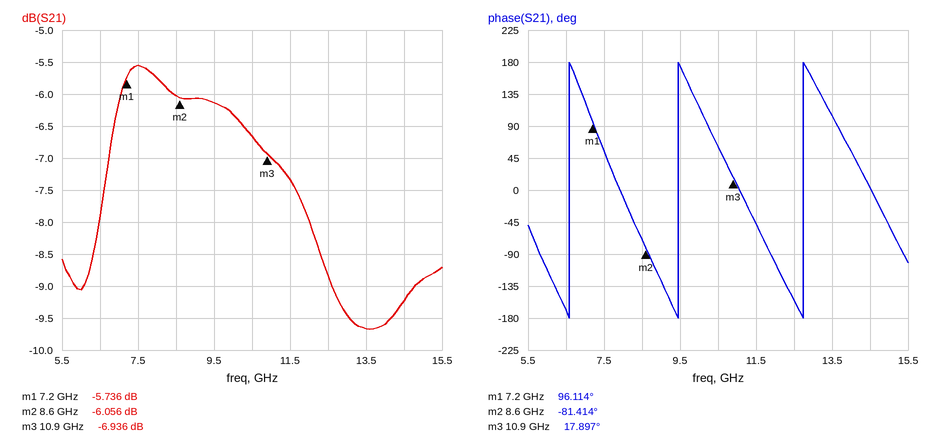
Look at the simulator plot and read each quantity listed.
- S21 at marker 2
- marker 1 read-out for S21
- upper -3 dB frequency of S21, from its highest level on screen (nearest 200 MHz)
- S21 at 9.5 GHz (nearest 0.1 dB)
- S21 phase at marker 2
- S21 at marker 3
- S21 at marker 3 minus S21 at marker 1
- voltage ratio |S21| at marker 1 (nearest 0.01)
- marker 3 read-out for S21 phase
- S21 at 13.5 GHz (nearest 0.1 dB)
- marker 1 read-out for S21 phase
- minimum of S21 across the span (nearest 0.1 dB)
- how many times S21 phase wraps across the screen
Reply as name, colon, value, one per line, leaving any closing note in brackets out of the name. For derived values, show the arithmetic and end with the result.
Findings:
S21 at marker 2: -6.056 dB
marker 1 read-out for S21: -5.736 dB
upper -3 dB frequency of S21, from its highest level on screen: 12.4 GHz
S21 at 9.5 GHz: -6.1 dB
S21 phase at marker 2: -81.414°
S21 at marker 3: -6.936 dB
S21 at marker 3 minus S21 at marker 1: -6.936 − (-5.736) = -1.200 dB
voltage ratio |S21| at marker 1: 10^(-5.736/20) ≈ 0.52
marker 3 read-out for S21 phase: 17.897°
S21 at 13.5 GHz: -9.7 dB
marker 1 read-out for S21 phase: 96.114°
minimum of S21 across the span: -9.7 dB
how many times S21 phase wraps across the screen: 3
